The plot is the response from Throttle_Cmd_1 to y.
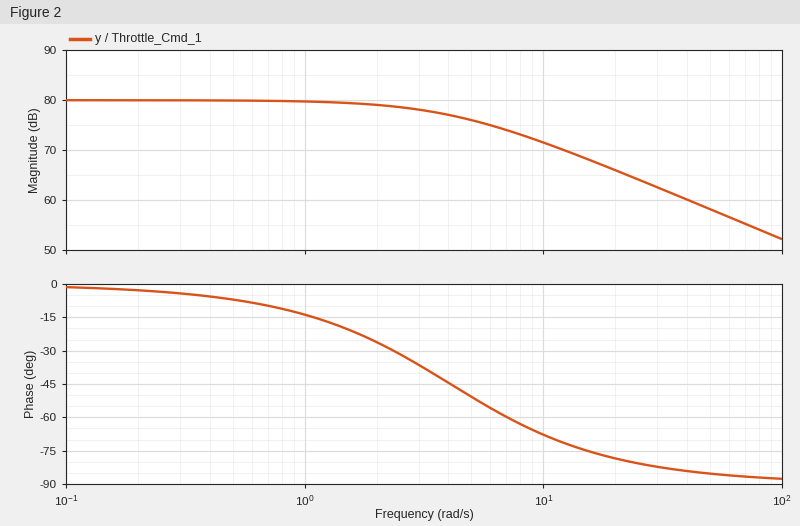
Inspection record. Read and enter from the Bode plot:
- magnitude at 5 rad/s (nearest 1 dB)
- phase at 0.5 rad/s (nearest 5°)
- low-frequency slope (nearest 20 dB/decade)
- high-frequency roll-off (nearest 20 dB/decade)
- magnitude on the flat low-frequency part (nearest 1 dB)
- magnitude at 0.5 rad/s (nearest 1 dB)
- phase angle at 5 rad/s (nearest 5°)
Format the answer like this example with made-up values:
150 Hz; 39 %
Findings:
76 dB; -5°; 0 dB/decade; -20 dB/decade; 80 dB; 80 dB; -50°
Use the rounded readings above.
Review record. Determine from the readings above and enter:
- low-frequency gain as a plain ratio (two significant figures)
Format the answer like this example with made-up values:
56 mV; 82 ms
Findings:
10000
